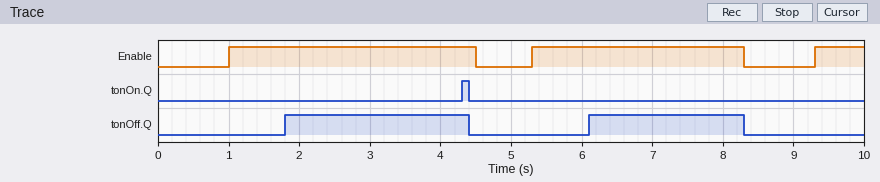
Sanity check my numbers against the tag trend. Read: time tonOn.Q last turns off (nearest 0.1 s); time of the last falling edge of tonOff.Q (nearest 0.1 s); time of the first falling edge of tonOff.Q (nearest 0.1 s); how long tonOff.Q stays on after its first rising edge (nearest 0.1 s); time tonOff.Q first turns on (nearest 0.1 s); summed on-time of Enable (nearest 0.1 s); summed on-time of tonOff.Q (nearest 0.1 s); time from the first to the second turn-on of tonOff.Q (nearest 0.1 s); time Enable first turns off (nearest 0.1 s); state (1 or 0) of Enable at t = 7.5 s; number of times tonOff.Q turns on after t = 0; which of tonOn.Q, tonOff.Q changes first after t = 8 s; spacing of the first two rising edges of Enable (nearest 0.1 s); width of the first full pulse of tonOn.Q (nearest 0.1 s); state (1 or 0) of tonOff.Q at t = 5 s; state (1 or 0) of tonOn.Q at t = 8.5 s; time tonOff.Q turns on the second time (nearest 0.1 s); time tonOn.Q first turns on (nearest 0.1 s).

4.4 s
8.3 s
4.4 s
2.6 s
1.8 s
7.2 s
4.8 s
4.3 s
4.5 s
1
2
tonOff.Q
4.3 s
0.1 s
0
0
6.1 s
4.3 s
